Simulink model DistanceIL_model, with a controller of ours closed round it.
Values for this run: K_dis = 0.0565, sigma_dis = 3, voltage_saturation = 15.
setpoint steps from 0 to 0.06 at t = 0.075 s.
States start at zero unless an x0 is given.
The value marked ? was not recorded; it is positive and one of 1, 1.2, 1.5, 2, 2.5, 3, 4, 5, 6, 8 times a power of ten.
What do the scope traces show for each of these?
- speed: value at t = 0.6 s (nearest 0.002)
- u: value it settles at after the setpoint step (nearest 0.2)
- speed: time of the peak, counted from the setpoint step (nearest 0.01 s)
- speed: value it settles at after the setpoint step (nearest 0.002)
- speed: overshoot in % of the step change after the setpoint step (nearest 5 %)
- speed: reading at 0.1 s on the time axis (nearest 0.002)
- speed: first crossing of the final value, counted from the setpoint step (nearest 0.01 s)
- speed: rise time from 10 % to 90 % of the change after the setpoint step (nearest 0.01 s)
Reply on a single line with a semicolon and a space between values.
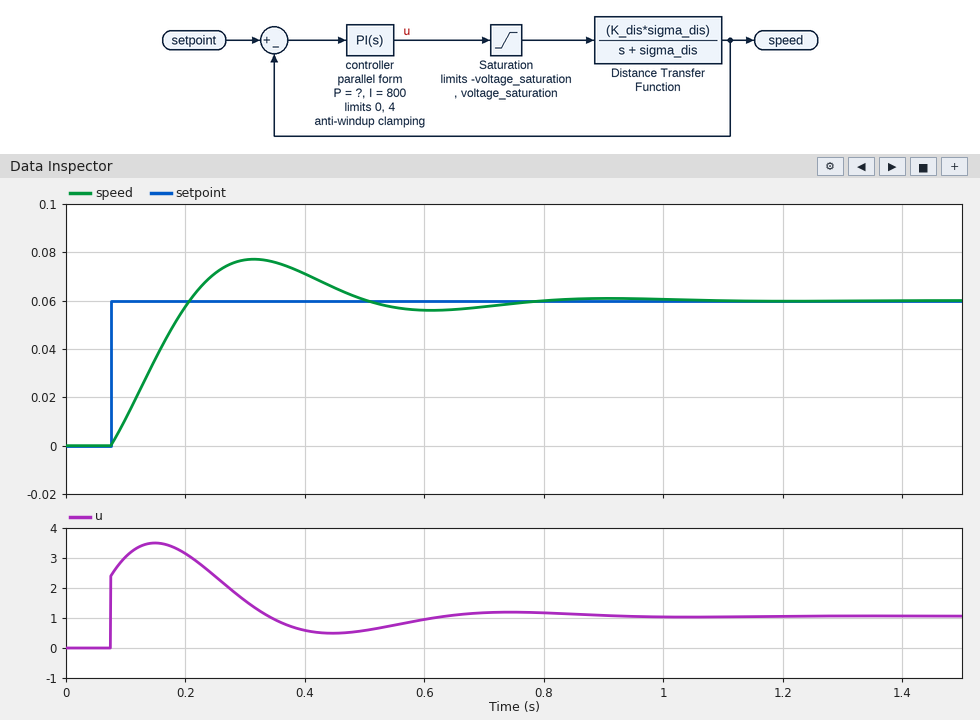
0.056; 1.0; 0.24 s; 0.060; 30 %; 0.012; 0.13 s; 0.10 s
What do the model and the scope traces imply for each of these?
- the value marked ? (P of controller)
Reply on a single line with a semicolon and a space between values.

40
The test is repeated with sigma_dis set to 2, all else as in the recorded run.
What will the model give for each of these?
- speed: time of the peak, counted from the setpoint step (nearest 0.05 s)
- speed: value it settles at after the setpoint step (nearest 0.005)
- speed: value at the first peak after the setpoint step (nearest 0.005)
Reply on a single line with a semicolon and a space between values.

0.30 s; 0.060; 0.080
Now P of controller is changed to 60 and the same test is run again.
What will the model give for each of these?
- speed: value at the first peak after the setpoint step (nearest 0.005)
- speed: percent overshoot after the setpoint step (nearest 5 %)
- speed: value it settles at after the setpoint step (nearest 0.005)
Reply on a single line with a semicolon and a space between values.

0.070; 20 %; 0.060
